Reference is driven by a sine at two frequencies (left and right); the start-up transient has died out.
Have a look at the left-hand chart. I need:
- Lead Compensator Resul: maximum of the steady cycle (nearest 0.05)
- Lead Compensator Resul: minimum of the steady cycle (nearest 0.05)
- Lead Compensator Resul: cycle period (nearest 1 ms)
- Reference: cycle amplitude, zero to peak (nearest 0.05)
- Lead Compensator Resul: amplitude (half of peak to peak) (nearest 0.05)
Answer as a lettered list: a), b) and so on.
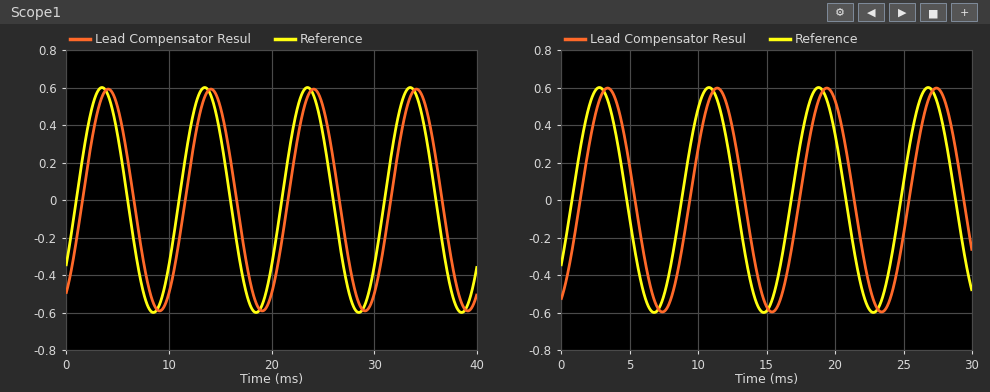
a) 0.60
b) -0.60
c) 10 ms
d) 0.60
e) 0.60
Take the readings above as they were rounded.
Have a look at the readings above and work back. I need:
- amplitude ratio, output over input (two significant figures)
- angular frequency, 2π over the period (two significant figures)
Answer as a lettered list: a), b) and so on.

a) 1.0
b) 0.63 rad/ms
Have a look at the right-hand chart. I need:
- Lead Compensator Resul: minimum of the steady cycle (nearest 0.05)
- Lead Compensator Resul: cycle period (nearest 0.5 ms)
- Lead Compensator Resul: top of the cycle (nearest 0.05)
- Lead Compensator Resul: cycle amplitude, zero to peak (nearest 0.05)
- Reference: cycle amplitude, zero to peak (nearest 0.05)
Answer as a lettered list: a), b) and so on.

a) -0.60
b) 8.0 ms
c) 0.60
d) 0.60
e) 0.60
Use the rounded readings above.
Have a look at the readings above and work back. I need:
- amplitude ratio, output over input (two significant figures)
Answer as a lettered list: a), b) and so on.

a) 1.0
